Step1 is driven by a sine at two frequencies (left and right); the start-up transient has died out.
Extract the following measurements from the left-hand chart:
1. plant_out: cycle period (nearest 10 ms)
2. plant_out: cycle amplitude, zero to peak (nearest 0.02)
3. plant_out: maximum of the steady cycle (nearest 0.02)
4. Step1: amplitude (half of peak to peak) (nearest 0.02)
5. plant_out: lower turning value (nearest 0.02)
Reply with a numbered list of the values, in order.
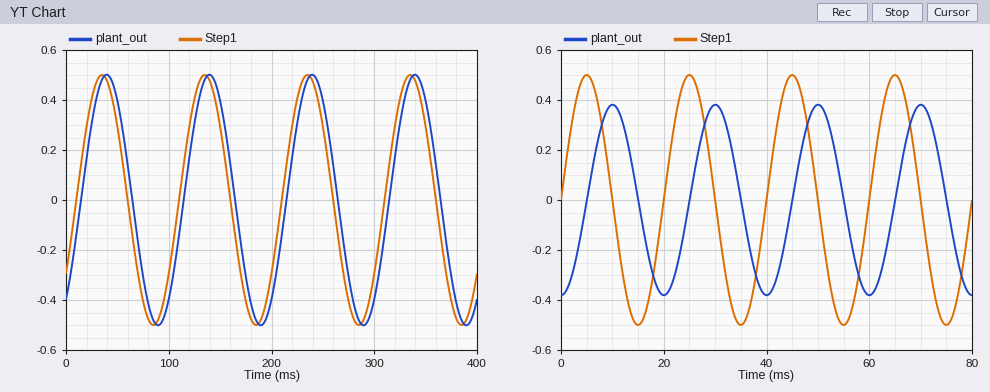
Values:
1. 100 ms
2. 0.50
3. 0.50
4. 0.50
5. -0.50
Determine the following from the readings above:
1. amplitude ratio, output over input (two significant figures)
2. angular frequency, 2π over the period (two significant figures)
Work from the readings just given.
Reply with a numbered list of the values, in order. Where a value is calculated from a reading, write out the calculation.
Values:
1. 0.5 / 0.5 = 1.0
2. 2π / 100 = 0.063 rad/ms
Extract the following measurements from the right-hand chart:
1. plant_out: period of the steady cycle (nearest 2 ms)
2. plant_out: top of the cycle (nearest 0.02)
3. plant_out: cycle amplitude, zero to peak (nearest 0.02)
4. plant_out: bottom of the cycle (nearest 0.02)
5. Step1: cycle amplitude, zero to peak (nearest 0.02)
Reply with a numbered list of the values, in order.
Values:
1. 20 ms
2. 0.38
3. 0.38
4. -0.38
5. 0.50
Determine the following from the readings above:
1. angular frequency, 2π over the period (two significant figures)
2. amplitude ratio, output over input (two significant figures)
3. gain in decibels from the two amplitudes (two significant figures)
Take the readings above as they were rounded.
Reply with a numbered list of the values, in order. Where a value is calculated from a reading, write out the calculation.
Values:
1. 2π / 20 = 0.31 rad/ms
2. 0.38 / 0.5 = 0.76
3. 20 log10(0.38 / 0.5) = -2.4 dB
